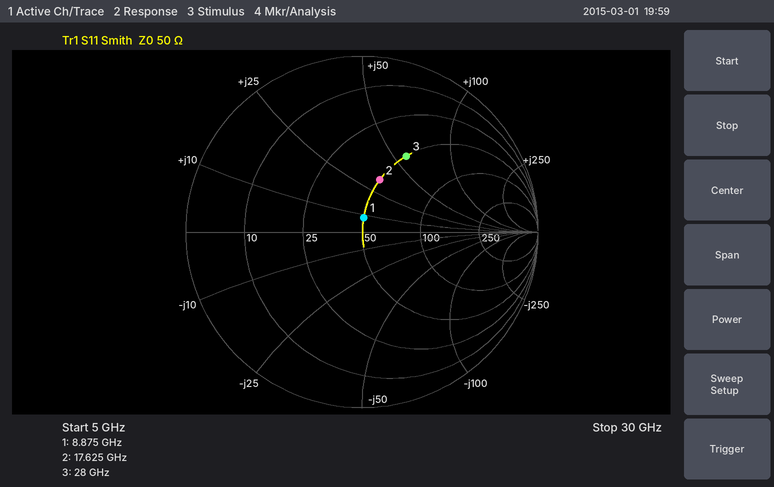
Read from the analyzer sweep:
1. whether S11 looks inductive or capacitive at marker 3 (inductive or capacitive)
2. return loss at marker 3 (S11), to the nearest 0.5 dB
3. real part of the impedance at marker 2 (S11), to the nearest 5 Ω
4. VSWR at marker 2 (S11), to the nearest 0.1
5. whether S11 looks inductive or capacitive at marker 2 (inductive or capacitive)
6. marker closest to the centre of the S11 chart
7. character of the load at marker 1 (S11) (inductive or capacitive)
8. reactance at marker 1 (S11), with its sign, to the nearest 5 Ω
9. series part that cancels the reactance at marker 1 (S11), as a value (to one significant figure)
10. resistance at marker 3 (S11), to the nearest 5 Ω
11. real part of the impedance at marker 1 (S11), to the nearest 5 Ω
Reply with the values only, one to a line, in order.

inductive
6.0 dB
50 Ω
1.9
inductive
marker 1
inductive
+10 Ω
2 pF
50 Ω
50 Ω
